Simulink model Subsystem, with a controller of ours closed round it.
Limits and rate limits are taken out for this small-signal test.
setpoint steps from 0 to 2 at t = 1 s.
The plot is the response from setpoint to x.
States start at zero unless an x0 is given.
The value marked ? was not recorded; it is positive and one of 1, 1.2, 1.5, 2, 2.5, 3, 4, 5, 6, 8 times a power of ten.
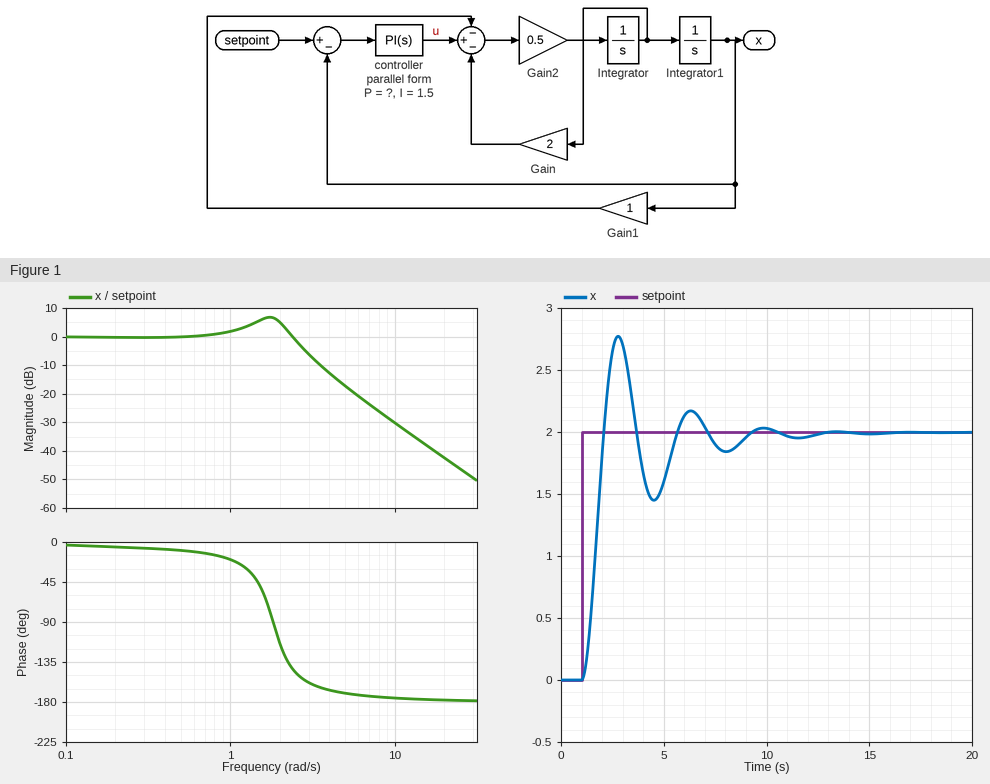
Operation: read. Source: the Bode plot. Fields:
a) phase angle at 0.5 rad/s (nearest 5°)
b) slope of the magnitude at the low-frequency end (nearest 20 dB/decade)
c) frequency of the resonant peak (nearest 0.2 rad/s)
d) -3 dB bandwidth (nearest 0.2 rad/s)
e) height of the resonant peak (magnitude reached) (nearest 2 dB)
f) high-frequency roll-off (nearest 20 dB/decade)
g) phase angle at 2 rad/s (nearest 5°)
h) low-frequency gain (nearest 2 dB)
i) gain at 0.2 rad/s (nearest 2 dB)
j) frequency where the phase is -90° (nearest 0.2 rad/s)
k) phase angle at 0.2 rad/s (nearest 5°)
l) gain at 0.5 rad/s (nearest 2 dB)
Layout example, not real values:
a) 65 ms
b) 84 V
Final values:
a) -10°
b) 0 dB/decade
c) 1.8 rad/s
d) 2.6 rad/s
e) 6 dB
f) -40 dB/decade
g) -115°
h) 0 dB
i) 0 dB
j) 1.8 rad/s
k) -5°
l) 0 dB
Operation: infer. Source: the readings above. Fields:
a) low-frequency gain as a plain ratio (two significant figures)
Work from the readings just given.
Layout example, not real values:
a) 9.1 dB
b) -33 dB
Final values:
a) 1.0
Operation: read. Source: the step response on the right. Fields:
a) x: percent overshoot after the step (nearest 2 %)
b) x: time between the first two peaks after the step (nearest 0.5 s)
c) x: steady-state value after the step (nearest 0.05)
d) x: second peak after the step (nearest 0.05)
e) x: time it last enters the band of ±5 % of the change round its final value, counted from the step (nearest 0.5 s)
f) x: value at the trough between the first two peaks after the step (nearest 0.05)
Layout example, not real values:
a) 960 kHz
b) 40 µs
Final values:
a) 38 %
b) 3.5 s
c) 2.00
d) 2.15
e) 7.5 s
f) 1.45
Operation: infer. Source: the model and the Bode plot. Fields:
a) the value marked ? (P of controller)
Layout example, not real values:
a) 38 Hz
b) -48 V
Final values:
a) 6
